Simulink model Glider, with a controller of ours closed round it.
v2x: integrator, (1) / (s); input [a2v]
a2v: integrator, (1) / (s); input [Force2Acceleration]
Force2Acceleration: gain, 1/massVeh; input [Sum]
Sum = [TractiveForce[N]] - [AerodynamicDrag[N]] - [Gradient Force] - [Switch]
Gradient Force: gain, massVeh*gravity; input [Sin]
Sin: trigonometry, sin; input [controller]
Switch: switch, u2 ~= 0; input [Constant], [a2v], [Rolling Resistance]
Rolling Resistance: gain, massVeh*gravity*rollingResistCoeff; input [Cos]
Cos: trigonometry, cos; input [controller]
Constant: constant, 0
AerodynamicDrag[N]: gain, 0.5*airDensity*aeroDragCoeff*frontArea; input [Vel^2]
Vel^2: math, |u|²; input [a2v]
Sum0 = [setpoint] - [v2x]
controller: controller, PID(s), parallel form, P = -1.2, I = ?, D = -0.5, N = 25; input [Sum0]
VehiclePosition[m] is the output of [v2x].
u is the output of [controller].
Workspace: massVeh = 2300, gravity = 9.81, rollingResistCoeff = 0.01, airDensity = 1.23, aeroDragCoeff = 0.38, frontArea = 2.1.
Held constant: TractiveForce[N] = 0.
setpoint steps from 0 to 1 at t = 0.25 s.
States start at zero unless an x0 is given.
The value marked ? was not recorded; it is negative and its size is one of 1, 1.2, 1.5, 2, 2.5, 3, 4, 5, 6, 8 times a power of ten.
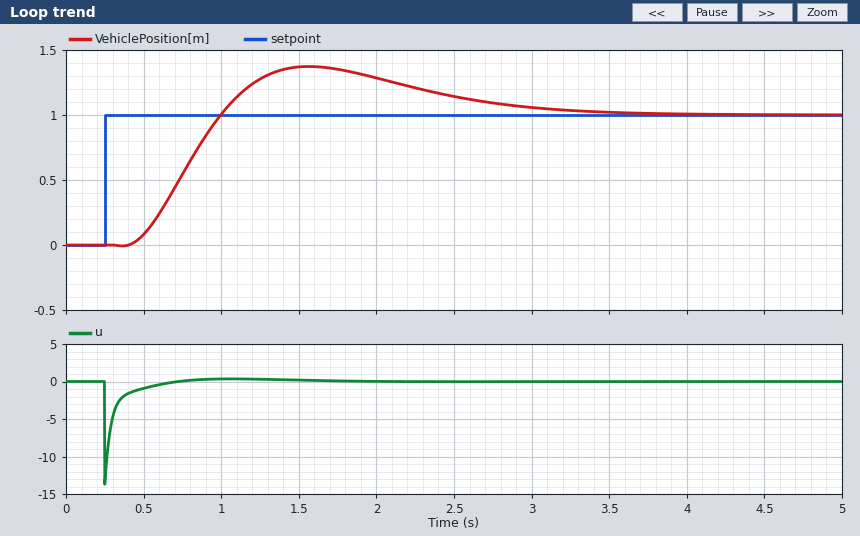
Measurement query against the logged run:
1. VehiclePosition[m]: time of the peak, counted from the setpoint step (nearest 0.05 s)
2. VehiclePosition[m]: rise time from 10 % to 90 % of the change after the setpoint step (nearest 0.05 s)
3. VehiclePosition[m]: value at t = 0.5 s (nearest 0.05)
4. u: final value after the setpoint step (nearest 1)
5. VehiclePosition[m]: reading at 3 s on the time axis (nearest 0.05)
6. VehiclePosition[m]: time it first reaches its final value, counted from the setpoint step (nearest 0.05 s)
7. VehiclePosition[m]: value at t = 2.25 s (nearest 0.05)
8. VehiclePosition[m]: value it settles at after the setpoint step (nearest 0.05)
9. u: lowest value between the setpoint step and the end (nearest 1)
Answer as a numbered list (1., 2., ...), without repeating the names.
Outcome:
1. 1.30 s
2. 0.40 s
3. 0.10
4. 0
5. 1.05
6. 0.75 s
7. 1.20
8. 1.00
9. -14
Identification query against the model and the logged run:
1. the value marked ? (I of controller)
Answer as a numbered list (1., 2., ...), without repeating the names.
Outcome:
1. -1
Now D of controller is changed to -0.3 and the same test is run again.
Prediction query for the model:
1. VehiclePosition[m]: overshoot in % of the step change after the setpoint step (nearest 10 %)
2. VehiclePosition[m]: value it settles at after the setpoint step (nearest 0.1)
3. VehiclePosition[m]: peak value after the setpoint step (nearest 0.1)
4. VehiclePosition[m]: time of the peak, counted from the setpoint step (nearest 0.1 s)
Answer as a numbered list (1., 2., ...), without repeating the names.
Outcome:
1. 60 %
2. 1.0
3. 1.6
4. 1.1 s
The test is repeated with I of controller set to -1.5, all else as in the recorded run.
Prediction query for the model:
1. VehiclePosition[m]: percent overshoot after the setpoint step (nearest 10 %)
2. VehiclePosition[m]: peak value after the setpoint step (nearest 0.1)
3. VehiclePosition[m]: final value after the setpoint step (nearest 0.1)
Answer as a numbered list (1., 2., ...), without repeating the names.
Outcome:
1. 50 %
2. 1.5
3. 1.0
